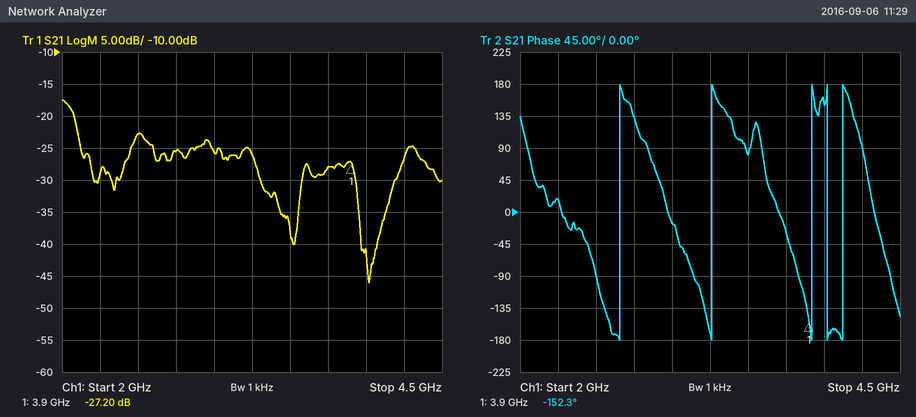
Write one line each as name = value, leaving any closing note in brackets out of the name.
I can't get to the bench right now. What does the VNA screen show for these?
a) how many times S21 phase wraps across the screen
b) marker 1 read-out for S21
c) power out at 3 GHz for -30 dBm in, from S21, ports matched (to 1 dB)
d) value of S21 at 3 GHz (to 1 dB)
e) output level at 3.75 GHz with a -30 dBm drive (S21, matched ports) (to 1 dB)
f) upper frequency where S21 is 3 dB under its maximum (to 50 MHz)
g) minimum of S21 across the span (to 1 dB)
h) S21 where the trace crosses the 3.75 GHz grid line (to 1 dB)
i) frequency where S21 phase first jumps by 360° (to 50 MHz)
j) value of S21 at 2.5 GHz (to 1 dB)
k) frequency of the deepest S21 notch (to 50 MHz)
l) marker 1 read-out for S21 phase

how many times S21 phase wraps across the screen = 5
marker 1 read-out for S21 = -27.20 dB
power out at 3 GHz for -30 dBm in, from S21, ports matched = -56 dBm
value of S21 at 3 GHz = -26 dB
output level at 3.75 GHz with a -30 dBm drive (S21, matched ports) = -58 dBm
upper frequency where S21 is 3 dB under its maximum = 2.10 GHz
minimum of S21 across the span = -46 dB
S21 where the trace crosses the 3.75 GHz grid line = -28 dB
frequency where S21 phase first jumps by 360° = 2.65 GHz
value of S21 at 2.5 GHz = -23 dB
frequency of the deepest S21 notch = 4.00 GHz
marker 1 read-out for S21 phase = -152.3°
